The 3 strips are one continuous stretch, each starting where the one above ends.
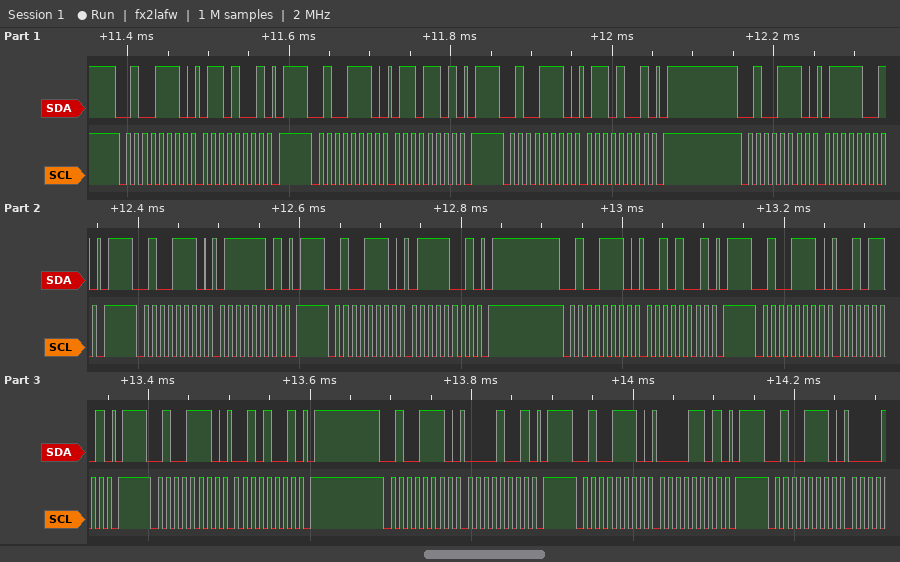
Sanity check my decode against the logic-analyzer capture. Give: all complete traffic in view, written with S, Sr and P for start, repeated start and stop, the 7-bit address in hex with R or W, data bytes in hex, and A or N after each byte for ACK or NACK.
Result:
S 27W A 69 A P S 27W A 6D A P S 27W A 69 A P S 27W A 79 A P S 27W A 7D A P S 27W A 79 A P S 27W A 29 A P S 27W A 2D A P S 27W A 29 A P S 27W A 09 A P S 27W A 0D A P S 27W A
